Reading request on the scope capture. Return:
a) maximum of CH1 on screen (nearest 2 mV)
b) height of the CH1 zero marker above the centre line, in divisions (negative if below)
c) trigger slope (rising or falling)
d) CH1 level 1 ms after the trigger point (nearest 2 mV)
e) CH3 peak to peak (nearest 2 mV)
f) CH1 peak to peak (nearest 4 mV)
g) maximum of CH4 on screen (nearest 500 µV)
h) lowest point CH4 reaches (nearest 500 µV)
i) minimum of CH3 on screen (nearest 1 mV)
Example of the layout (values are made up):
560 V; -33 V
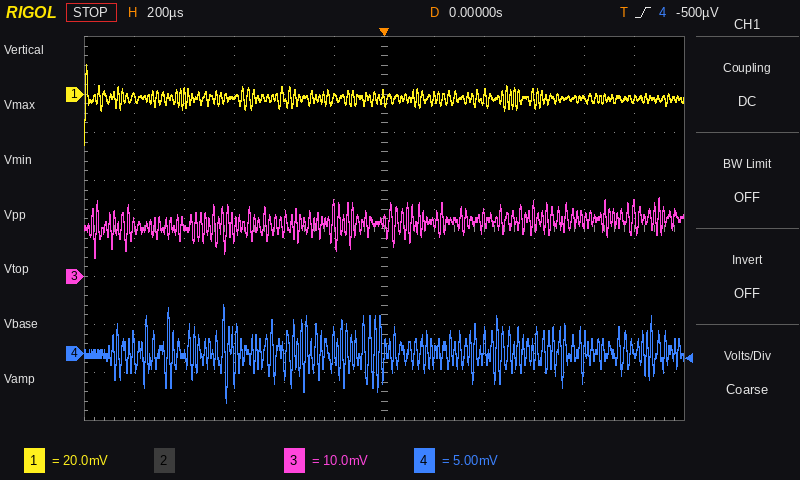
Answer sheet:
12 mV; +2.8 div; rising; -2 mV; 12 mV; 32 mV; 5.0 mV; -5.0 mV; 4 mV
